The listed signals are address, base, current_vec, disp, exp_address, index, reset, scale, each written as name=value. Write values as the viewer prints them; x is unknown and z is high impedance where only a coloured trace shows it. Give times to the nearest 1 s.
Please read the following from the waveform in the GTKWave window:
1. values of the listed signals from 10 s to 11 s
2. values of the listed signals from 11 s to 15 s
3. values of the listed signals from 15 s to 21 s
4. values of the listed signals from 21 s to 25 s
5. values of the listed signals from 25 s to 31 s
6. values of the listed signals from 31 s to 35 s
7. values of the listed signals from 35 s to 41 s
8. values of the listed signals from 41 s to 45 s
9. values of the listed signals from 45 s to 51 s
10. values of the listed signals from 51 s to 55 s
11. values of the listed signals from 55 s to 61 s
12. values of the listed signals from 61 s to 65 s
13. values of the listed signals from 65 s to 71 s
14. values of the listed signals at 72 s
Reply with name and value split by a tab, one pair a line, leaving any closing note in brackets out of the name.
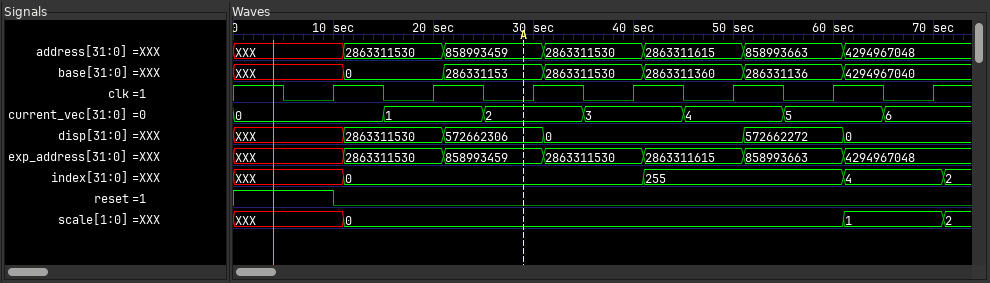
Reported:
values of the listed signals from 10 s to 11 s	address=XXX, base=XXX, current_vec=0, disp=XXX, exp_address=XXX, index=XXX, reset=0, scale=XXX
values of the listed signals from 11 s to 15 s	address=2863311530, base=0, current_vec=0, disp=2863311530, exp_address=2863311530, index=0, reset=0, scale=0
values of the listed signals from 15 s to 21 s	address=2863311530, base=0, current_vec=1, disp=2863311530, exp_address=2863311530, index=0, reset=0, scale=0
values of the listed signals from 21 s to 25 s	address=858993459, base=286331153, current_vec=1, disp=572662306, exp_address=858993459, index=0, reset=0, scale=0
values of the listed signals from 25 s to 31 s	address=858993459, base=286331153, current_vec=2, disp=572662306, exp_address=858993459, index=0, reset=0, scale=0
values of the listed signals from 31 s to 35 s	address=2863311530, base=2863311530, current_vec=2, disp=0, exp_address=2863311530, index=0, reset=0, scale=0
values of the listed signals from 35 s to 41 s	address=2863311530, base=2863311530, current_vec=3, disp=0, exp_address=2863311530, index=0, reset=0, scale=0
values of the listed signals from 41 s to 45 s	address=2863311615, base=2863311360, current_vec=3, disp=0, exp_address=2863311615, index=255, reset=0, scale=0
values of the listed signals from 45 s to 51 s	address=2863311615, base=2863311360, current_vec=4, disp=0, exp_address=2863311615, index=255, reset=0, scale=0
values of the listed signals from 51 s to 55 s	address=858993663, base=286331136, current_vec=4, disp=572662272, exp_address=858993663, index=255, reset=0, scale=0
values of the listed signals from 55 s to 61 s	address=858993663, base=286331136, current_vec=5, disp=572662272, exp_address=858993663, index=255, reset=0, scale=0
values of the listed signals from 61 s to 65 s	address=4294967048, base=4294967040, current_vec=5, disp=0, exp_address=4294967048, index=4, reset=0, scale=1
values of the listed signals from 65 s to 71 s	address=4294967048, base=4294967040, current_vec=6, disp=0, exp_address=4294967048, index=4, reset=0, scale=1
values of the listed signals at 72 s	address=4294967048, base=4294967040, current_vec=6, disp=0, exp_address=4294967048, index=2, reset=0, scale=2
